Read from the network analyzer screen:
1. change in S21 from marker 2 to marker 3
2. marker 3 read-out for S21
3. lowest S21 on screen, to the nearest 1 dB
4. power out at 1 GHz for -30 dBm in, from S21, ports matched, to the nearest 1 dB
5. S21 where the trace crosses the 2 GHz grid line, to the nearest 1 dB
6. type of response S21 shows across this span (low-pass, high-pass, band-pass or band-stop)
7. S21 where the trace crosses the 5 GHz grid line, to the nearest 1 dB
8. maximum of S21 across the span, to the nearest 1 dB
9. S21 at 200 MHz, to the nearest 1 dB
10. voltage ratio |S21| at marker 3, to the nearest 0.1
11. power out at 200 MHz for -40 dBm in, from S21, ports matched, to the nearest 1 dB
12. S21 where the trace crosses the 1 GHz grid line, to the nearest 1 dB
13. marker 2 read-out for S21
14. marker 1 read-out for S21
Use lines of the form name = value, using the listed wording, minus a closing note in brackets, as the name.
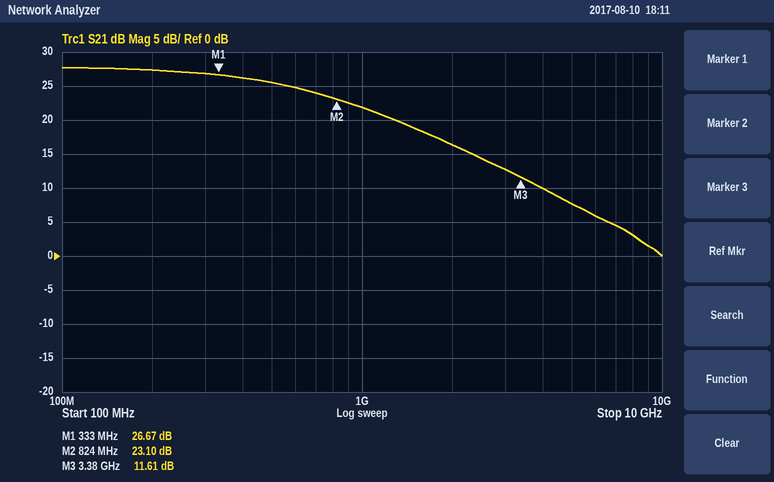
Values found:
change in S21 from marker 2 to marker 3 = -11.49 dB
marker 3 read-out for S21 = 11.61 dB
lowest S21 on screen, to the nearest 1 dB = 0 dB
power out at 1 GHz for -30 dBm in, from S21, ports matched, to the nearest 1 dB = -8 dBm
S21 where the trace crosses the 2 GHz grid line, to the nearest 1 dB = 16 dB
type of response S21 shows across this span = low-pass
S21 where the trace crosses the 5 GHz grid line, to the nearest 1 dB = 8 dB
maximum of S21 across the span, to the nearest 1 dB = 28 dB
S21 at 200 MHz, to the nearest 1 dB = 27 dB
voltage ratio |S21| at marker 3, to the nearest 0.1 = 3.8
power out at 200 MHz for -40 dBm in, from S21, ports matched, to the nearest 1 dB = -13 dBm
S21 where the trace crosses the 1 GHz grid line, to the nearest 1 dB = 22 dB
marker 2 read-out for S21 = 23.10 dB
marker 1 read-out for S21 = 26.67 dB
